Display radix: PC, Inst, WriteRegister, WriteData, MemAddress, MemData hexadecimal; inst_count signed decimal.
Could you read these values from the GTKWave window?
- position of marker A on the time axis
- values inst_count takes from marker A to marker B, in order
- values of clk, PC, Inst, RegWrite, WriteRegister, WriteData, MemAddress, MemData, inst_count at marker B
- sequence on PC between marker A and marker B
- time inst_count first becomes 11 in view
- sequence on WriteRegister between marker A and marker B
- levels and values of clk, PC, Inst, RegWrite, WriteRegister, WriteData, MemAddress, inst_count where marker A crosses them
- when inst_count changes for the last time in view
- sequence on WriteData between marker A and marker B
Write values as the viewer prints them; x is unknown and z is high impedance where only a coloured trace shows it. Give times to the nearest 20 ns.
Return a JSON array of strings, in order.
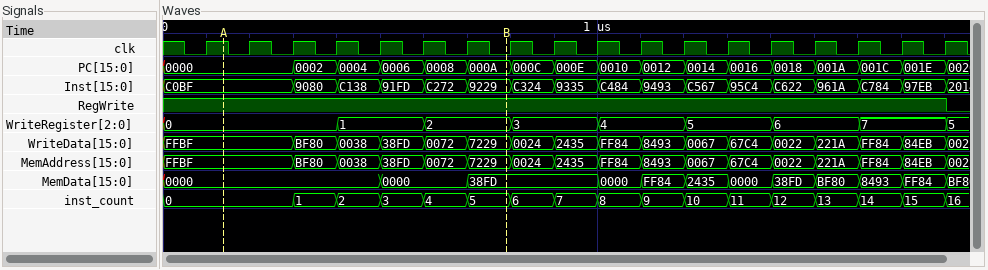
["140 ns", "0, 1, 2, 3, 4, 5", "clk=0, PC=000A, Inst=9229, RegWrite=1, WriteRegister=2, WriteData=7229, MemAddress=7229, MemData=38FD, inst_count=5", "0000, 0002, 0004, 0006, 0008, 000A", "1300 ns", "0, 1, 2", "clk=1, PC=0000, Inst=C0BF, RegWrite=1, WriteRegister=0, WriteData=FFBF, MemAddress=FFBF, inst_count=0", "1800 ns", "FFBF, BF80, 0038, 38FD, 0072, 7229"]
